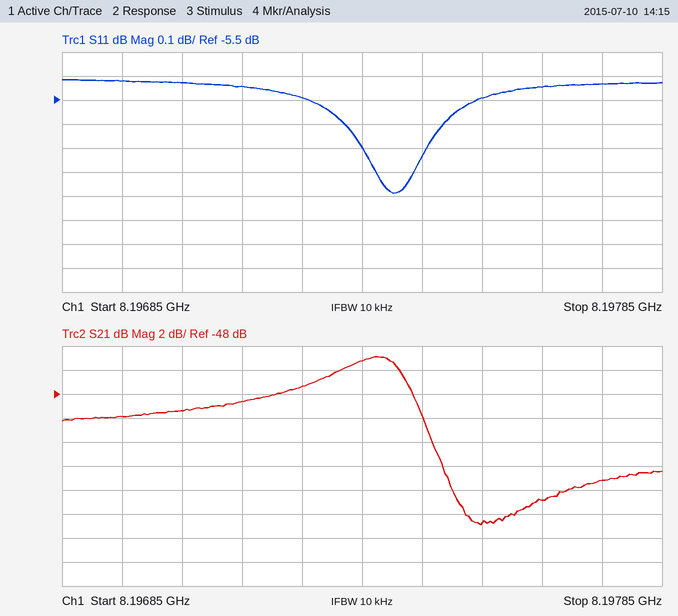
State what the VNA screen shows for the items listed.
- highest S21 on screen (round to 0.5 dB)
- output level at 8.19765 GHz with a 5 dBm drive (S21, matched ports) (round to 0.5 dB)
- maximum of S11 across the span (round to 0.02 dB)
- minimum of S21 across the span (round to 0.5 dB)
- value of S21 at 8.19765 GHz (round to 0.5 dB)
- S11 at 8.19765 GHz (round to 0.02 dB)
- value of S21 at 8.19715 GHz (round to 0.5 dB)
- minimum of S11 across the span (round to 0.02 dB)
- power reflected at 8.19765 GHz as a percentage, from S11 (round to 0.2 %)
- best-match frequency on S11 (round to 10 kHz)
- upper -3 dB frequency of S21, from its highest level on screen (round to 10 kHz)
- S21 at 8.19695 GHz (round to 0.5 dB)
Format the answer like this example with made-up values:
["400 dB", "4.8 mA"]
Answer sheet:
["-45.0 dB", "-52.0 dBm", "-5.42 dB", "-59.0 dB", "-57.0 dB", "-5.44 dB", "-48.5 dB", "-5.88 dB", "28.6 %", "8.19740 GHz", "8.19743 GHz", "-50.0 dB"]
